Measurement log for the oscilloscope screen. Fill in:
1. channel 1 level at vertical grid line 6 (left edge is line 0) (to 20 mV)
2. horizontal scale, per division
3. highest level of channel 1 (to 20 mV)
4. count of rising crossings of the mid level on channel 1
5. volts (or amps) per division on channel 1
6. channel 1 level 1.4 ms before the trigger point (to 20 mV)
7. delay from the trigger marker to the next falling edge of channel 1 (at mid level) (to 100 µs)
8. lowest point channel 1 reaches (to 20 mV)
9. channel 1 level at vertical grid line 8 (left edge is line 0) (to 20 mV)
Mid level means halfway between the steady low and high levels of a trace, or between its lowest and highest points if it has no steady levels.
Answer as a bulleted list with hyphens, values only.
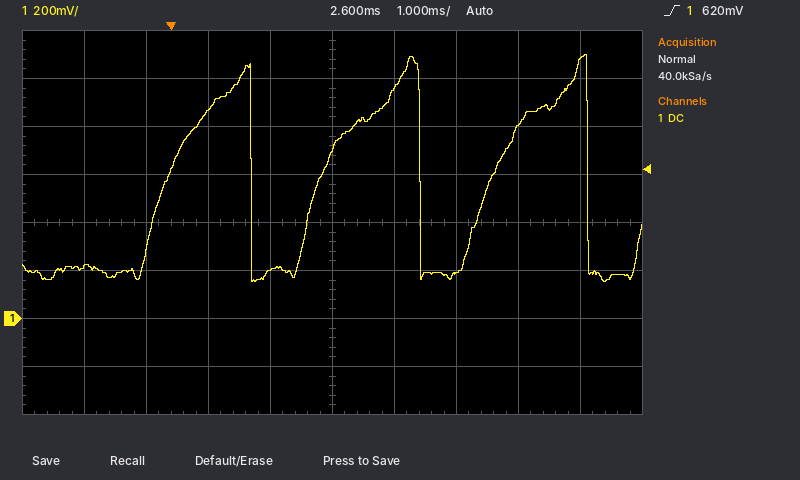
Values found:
- 960 mV
- 1 ms
- 1.10 V
- 3
- 200 mV
- 220 mV
- 1.3 ms
- 160 mV
- 800 mV
